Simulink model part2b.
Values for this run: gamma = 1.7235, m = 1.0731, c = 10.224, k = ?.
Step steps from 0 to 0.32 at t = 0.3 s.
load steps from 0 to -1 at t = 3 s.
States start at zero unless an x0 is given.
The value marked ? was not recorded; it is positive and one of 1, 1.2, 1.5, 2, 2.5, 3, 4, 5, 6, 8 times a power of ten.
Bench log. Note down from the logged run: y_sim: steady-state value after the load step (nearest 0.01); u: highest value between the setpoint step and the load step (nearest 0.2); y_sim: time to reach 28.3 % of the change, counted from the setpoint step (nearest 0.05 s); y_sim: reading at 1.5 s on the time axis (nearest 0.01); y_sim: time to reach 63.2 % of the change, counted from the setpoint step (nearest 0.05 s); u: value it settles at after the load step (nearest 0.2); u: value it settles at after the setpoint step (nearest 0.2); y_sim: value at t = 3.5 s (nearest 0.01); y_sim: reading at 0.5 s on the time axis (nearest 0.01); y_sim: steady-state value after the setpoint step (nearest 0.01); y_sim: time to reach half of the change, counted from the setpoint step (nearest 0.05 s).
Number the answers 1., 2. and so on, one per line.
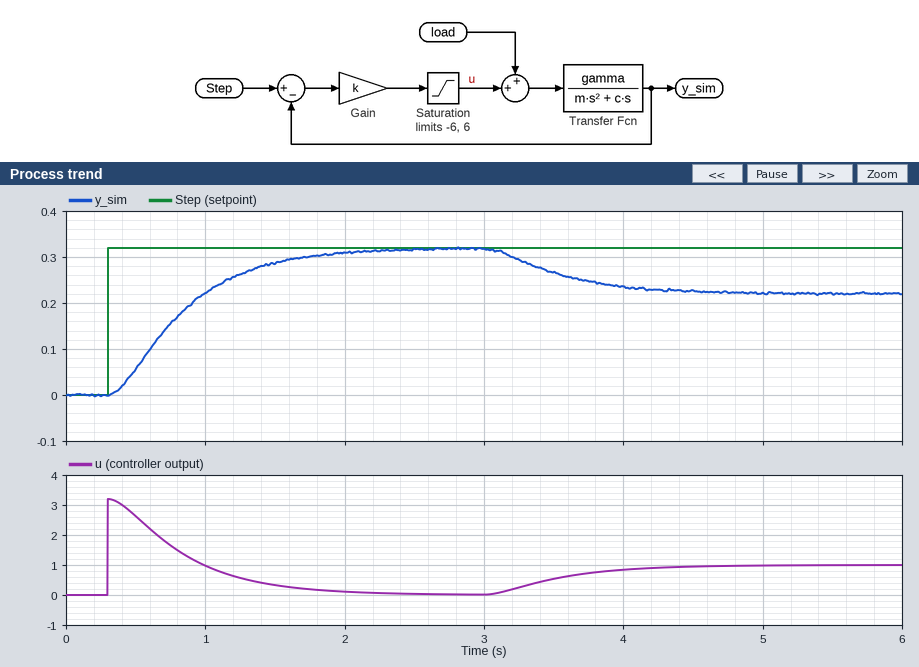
1. 0.22
2. 3.2
3. 0.30 s
4. 0.29
5. 0.60 s
6. 1.0
7. 0.0
8. 0.27
9. 0.06
10. 0.32
11. 0.45 s
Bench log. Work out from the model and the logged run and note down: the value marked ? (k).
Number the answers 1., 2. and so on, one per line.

1. 10
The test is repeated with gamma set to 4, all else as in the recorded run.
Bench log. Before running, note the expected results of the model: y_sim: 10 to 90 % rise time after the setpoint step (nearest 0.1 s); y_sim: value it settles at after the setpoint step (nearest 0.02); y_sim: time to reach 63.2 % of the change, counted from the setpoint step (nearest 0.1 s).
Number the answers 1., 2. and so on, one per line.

1. 0.4 s
2. 0.32
3. 0.3 s
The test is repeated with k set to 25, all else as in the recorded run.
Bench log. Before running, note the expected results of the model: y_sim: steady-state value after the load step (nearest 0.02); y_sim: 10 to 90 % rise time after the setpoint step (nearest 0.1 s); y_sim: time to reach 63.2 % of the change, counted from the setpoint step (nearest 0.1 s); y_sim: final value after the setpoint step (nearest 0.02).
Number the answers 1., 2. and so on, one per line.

1. 0.28
2. 0.4 s
3. 0.3 s
4. 0.32
